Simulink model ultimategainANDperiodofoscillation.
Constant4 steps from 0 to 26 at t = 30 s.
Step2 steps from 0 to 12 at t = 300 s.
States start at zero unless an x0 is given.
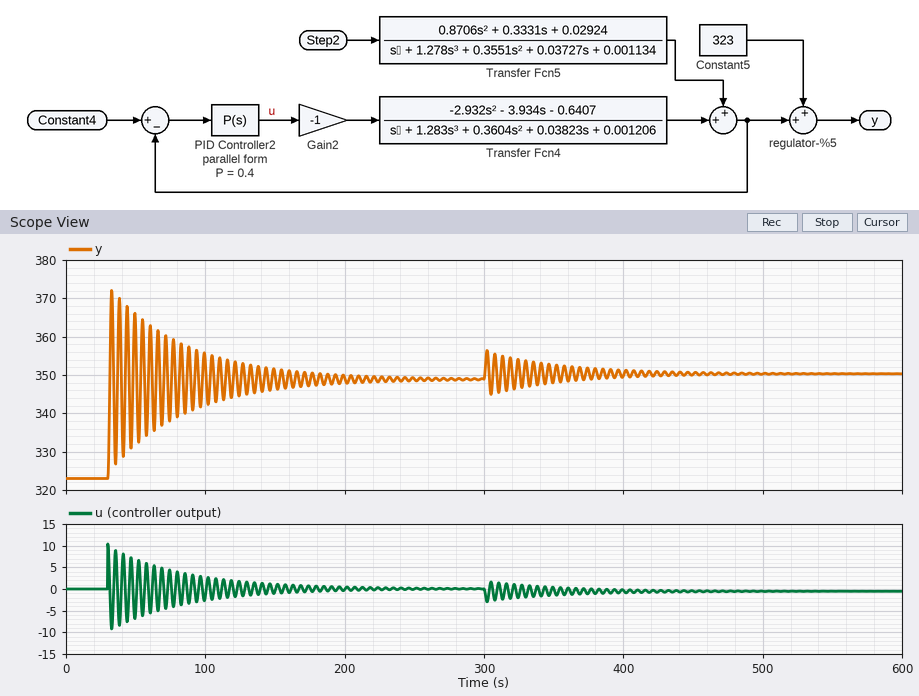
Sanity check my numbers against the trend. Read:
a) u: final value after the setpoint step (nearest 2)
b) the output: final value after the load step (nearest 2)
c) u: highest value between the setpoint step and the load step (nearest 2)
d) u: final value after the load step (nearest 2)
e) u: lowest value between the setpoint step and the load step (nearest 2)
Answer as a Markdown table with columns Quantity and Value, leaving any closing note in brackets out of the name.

| Quantity | Value |
|---|---|
| u: final value after the setpoint step | 0 |
| the output: final value after the load step | 350 |
| u: highest value between the setpoint step and the load step | 10 |
| u: final value after the load step | 0 |
| u: lowest value between the setpoint step and the load step | -10 |
